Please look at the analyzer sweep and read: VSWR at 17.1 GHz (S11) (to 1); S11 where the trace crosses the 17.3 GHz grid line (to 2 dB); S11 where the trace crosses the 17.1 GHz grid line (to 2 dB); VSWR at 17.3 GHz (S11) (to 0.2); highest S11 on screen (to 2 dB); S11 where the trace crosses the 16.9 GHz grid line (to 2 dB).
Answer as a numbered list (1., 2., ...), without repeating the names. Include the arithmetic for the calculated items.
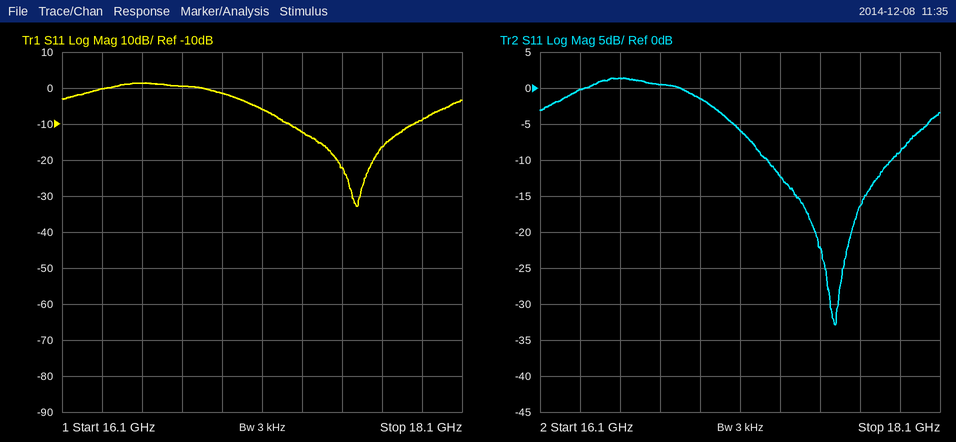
1. |Γ| = 10^(-6/20) = 0.5012; VSWR = (1 + 0.5012)/(1 − 0.5012) ≈ 3
2. -12 dB
3. -6 dB
4. |Γ| = 10^(-12/20) = 0.2512; VSWR = (1 + 0.2512)/(1 − 0.2512) ≈ 1.67, so 1.6 to the nearest 0.2
5. 2 dB
6. -2 dB
